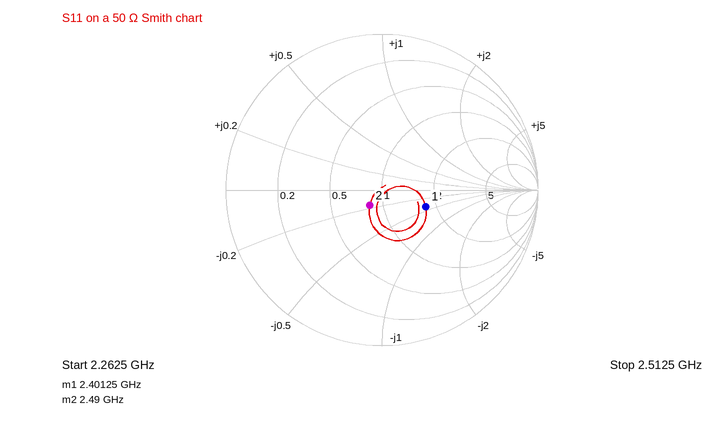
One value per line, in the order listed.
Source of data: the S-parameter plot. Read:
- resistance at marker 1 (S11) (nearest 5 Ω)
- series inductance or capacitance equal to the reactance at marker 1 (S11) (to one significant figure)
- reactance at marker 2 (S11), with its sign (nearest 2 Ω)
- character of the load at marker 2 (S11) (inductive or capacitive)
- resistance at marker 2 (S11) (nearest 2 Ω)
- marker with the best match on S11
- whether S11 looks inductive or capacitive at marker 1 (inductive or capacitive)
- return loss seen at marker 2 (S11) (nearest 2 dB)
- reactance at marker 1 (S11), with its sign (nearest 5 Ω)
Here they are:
85 Ω
3 pF
-8 Ω
capacitive
42 Ω
marker 2
capacitive
18 dB
-20 Ω
